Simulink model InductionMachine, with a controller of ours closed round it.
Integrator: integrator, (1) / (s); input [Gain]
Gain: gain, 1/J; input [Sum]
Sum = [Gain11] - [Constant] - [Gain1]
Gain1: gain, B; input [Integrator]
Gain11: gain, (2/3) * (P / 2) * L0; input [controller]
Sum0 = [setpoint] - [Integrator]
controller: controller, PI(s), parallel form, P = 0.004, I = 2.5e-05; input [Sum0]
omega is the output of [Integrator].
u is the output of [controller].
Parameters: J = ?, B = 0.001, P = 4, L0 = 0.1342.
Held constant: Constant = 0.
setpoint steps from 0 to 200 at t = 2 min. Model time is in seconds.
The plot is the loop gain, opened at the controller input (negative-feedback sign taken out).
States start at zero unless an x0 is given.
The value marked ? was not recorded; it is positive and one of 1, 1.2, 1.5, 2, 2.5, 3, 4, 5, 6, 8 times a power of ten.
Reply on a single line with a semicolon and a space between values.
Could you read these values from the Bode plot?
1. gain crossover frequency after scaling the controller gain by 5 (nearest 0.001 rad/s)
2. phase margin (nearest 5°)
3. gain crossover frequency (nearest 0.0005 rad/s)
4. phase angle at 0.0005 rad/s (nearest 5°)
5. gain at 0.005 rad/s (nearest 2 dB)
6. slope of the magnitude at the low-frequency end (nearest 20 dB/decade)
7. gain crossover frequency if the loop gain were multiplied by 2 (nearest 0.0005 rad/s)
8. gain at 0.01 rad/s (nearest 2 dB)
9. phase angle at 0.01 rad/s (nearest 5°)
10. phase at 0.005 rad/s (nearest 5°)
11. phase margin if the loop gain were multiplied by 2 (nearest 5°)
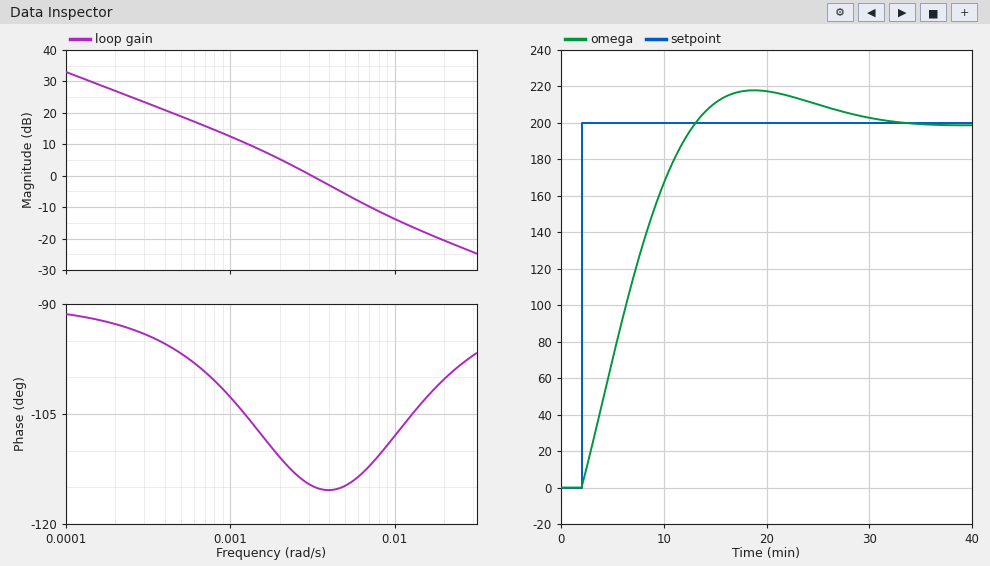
0.010 rad/s; 65°; 0.0030 rad/s; -95°; -6 dB; -20 dB/decade; 0.0050 rad/s; -14 dB; -110°; -115°; 65°
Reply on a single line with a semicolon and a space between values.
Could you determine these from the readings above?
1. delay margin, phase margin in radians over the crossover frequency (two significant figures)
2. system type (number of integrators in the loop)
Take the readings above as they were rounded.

380 s; 1
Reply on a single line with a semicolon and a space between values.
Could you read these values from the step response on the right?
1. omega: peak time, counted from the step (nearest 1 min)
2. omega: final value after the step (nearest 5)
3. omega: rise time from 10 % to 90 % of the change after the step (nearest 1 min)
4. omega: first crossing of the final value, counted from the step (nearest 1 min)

17 min; 200; 8 min; 11 min
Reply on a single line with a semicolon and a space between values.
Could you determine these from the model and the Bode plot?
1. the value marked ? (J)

0.4
